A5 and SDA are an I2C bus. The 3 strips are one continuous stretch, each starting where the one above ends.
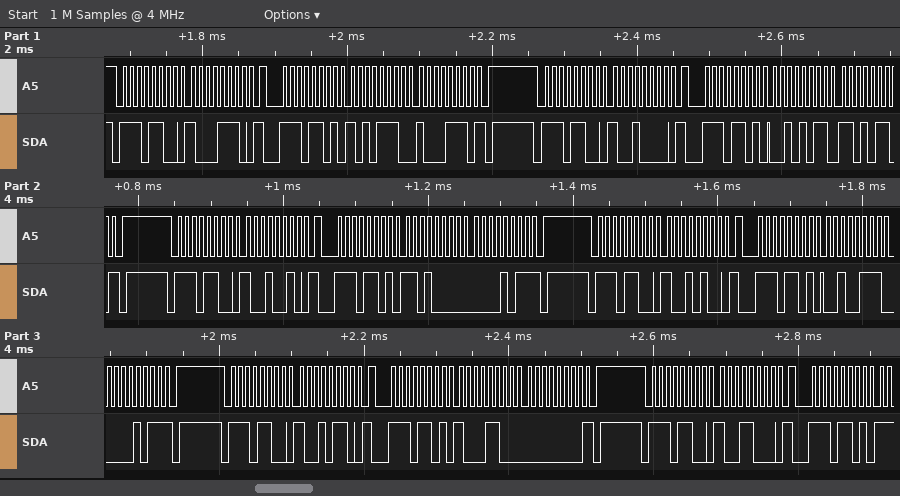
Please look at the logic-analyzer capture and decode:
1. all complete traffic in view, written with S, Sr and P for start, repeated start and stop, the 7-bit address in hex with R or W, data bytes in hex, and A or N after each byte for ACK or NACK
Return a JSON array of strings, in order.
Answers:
["S 76W A 8E A Sr 76R A AE A 8E N P S 76W A 90 A Sr 76R A 2B A D6 N P S 76W A 92 A Sr 76R A D0 A 0B N P S 76W A 94 A Sr 76R A 27 A 0B N P S 76W A 96 A Sr 76R A 8C A 00 N P S 76W A 98 A Sr 76R A"]
